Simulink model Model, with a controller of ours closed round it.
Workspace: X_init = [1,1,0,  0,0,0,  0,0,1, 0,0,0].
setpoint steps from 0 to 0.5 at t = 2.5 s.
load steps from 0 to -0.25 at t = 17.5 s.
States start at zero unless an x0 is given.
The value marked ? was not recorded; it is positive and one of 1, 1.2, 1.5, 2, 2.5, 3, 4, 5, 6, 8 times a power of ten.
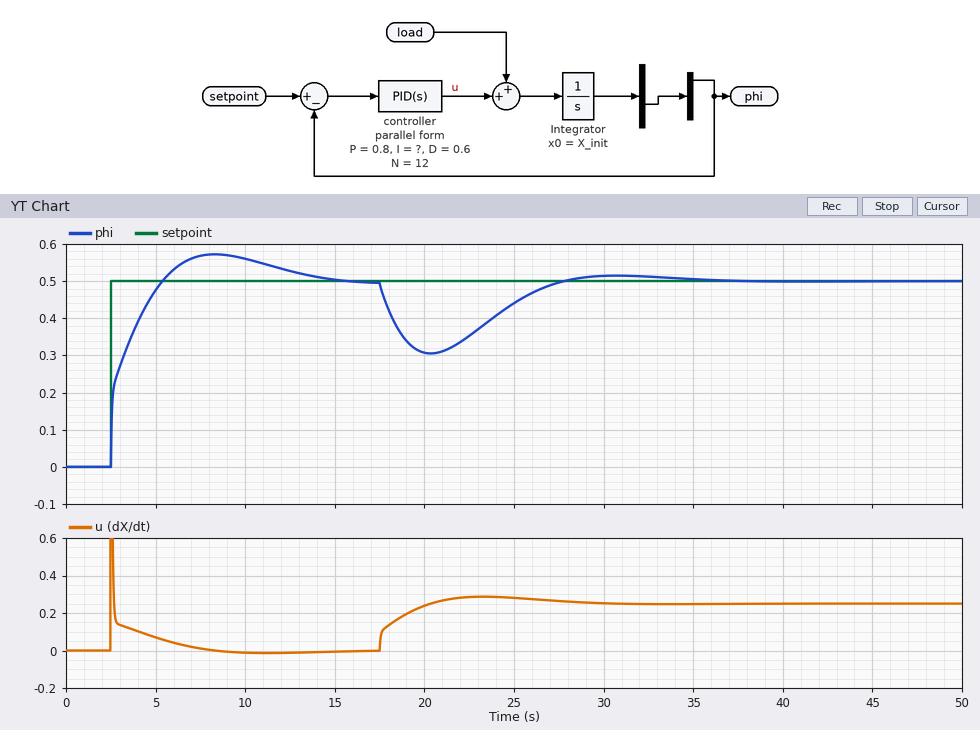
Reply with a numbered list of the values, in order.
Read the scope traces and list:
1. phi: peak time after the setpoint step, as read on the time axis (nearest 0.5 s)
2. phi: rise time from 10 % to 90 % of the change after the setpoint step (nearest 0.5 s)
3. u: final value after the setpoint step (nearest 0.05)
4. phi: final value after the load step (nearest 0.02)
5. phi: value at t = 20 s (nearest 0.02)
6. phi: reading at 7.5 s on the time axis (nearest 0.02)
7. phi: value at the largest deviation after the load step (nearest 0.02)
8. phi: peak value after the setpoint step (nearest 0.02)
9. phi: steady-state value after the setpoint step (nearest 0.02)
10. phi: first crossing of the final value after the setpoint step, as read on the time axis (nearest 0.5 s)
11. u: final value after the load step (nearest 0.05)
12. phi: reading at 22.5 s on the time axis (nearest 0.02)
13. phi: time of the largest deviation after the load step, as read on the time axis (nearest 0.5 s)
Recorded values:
1. 8.5 s
2. 2.0 s
3. 0.00
4. 0.50
5. 0.30
6. 0.56
7. 0.30
8. 0.58
9. 0.50
10. 5.5 s
11. 0.25
12. 0.36
13. 20.5 s
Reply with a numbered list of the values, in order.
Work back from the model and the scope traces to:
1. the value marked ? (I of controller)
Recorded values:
1. 0.25
